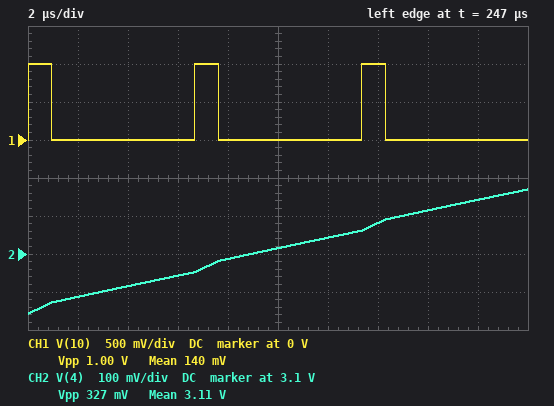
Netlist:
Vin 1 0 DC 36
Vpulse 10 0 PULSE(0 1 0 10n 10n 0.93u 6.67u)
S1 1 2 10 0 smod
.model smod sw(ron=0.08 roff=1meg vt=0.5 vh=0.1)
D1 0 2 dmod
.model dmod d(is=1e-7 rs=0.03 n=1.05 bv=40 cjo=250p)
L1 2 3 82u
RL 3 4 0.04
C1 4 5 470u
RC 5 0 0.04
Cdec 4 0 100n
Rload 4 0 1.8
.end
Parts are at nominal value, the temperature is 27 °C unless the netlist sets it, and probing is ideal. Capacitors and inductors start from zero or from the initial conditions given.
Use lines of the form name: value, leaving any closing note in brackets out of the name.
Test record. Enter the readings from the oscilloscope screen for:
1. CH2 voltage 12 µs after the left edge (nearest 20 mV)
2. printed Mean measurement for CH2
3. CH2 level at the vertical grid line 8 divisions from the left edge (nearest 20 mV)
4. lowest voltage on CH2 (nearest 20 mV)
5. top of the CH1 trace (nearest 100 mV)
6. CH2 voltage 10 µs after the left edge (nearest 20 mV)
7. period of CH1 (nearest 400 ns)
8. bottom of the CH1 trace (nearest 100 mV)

CH2 voltage 12 µs after the left edge: 3.14 V
printed Mean measurement for CH2: 3.11 V
CH2 level at the vertical grid line 8 divisions from the left edge: 3.22 V
lowest voltage on CH2: 2.94 V
top of the CH1 trace: 1.0 V
CH2 voltage 10 µs after the left edge: 3.12 V
period of CH1: 6.8 µs
bottom of the CH1 trace: 0 V
